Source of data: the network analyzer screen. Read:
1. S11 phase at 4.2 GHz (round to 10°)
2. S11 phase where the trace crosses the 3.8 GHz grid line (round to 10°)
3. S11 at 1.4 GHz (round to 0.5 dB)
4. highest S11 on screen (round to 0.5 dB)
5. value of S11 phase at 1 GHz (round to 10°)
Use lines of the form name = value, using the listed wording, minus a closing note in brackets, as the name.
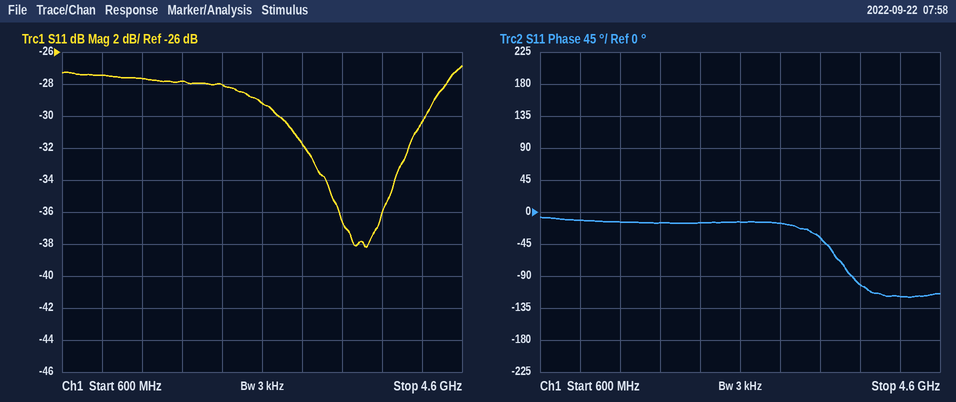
S11 phase at 4.2 GHz = -120°
S11 phase where the trace crosses the 3.8 GHz grid line = -100°
S11 at 1.4 GHz = -27.5 dB
highest S11 on screen = -27.0 dB
value of S11 phase at 1 GHz = -10°
